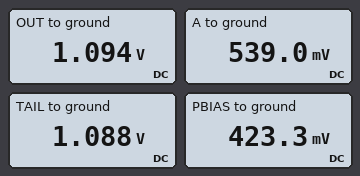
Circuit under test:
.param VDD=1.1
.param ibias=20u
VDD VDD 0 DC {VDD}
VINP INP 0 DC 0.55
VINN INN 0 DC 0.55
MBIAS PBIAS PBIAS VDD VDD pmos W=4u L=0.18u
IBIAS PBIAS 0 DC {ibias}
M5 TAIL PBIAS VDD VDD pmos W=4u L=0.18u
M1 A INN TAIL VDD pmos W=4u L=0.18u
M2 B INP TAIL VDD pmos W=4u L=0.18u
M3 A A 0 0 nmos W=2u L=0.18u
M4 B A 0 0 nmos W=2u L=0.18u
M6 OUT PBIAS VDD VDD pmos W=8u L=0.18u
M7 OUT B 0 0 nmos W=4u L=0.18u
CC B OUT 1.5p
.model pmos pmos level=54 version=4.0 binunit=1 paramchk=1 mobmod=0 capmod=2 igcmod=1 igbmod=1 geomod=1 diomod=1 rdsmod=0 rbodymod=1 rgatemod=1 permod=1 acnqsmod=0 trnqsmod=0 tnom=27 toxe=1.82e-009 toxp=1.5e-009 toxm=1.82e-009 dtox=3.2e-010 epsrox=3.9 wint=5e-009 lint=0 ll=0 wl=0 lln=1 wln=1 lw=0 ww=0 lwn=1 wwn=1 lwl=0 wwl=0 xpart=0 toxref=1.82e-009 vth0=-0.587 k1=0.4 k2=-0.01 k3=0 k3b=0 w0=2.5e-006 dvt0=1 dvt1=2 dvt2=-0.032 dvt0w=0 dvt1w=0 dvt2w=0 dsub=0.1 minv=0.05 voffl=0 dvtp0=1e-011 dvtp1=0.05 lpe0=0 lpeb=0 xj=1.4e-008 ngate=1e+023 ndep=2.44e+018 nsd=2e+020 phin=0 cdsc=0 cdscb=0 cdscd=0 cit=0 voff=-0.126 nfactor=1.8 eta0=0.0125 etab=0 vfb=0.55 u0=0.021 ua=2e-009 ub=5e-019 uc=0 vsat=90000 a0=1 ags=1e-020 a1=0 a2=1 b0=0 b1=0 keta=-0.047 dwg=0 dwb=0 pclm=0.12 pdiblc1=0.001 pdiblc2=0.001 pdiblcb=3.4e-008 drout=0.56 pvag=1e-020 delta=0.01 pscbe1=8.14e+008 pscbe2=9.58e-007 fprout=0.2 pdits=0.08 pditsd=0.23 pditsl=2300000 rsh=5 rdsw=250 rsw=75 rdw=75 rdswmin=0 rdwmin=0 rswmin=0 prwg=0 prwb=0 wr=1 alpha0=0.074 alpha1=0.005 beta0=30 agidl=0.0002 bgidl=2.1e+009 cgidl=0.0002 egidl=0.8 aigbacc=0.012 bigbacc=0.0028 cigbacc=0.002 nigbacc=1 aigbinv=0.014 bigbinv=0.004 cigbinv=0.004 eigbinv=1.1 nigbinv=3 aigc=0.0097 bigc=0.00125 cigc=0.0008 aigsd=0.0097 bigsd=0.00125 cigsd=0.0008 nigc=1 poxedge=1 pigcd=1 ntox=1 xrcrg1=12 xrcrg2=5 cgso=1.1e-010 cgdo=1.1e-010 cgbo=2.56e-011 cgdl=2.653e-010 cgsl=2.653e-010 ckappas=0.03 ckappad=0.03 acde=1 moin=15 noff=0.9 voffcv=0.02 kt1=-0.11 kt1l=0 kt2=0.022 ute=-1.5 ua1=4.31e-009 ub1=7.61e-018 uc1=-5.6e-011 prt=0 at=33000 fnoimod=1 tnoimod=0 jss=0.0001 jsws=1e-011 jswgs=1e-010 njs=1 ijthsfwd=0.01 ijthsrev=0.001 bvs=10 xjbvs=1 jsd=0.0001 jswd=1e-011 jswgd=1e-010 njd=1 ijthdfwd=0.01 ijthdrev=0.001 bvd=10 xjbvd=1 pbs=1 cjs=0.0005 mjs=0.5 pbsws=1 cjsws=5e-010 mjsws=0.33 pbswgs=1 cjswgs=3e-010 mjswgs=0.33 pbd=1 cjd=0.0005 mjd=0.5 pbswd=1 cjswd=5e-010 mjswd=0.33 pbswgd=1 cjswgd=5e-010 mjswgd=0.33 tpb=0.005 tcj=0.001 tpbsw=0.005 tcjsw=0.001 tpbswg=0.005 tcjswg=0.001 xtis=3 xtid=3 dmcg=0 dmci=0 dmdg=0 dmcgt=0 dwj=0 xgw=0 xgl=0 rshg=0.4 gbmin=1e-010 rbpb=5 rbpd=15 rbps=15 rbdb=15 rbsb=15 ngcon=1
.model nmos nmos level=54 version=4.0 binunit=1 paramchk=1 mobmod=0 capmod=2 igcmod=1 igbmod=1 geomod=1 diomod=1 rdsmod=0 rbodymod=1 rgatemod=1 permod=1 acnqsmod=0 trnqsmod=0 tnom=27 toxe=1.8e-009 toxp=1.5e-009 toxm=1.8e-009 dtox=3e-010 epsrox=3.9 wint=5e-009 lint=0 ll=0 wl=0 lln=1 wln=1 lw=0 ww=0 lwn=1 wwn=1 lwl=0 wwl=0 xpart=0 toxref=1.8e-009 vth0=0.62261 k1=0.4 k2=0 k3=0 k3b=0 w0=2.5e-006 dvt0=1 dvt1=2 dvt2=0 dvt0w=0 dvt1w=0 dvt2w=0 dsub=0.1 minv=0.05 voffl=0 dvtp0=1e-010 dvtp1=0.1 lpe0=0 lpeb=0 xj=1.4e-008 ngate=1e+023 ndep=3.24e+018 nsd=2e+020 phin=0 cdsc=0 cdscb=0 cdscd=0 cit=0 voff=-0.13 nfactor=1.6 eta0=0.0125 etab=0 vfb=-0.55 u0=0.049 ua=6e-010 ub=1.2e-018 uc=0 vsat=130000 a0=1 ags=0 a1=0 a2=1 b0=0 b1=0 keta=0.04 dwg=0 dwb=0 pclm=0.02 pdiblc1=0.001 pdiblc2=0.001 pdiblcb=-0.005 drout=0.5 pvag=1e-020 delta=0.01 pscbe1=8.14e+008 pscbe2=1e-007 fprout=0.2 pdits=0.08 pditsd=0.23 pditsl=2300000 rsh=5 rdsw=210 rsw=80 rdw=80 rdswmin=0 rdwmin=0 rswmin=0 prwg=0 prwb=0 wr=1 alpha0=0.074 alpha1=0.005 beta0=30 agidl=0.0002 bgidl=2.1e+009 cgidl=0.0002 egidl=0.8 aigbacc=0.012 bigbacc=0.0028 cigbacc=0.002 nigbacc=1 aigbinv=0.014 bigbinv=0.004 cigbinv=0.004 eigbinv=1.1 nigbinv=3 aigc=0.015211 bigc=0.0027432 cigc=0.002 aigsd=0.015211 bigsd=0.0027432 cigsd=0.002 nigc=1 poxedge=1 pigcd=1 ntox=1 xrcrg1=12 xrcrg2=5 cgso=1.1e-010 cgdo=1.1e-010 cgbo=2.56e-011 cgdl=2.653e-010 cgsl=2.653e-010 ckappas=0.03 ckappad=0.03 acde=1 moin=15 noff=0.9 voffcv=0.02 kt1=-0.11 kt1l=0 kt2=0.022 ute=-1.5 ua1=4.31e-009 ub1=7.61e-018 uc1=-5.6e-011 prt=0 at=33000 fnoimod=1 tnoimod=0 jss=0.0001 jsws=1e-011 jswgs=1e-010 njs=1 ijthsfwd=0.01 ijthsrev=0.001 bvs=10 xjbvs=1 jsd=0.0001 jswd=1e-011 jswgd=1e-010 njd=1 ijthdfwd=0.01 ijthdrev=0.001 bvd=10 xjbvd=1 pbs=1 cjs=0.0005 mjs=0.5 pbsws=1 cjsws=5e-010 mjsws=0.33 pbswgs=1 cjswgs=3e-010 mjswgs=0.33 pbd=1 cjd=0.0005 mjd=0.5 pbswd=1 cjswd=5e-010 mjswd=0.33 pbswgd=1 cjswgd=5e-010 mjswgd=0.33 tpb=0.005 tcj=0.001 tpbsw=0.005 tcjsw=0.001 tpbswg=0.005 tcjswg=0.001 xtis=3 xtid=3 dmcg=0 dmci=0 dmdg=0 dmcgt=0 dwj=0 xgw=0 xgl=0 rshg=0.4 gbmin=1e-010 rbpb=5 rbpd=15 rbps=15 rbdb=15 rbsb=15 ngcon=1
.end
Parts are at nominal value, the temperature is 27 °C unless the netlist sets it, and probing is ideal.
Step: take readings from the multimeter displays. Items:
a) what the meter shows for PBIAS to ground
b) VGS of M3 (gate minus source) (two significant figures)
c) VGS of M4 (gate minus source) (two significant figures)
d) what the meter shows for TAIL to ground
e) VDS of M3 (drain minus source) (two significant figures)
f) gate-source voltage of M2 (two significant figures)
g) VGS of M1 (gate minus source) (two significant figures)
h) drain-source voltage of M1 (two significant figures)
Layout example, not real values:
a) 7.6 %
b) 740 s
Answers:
a) 423.3 mV
b) 540 mV
c) 540 mV
d) 1.088 V
e) 540 mV
f) -540 mV
g) -540 mV
h) -550 mV
